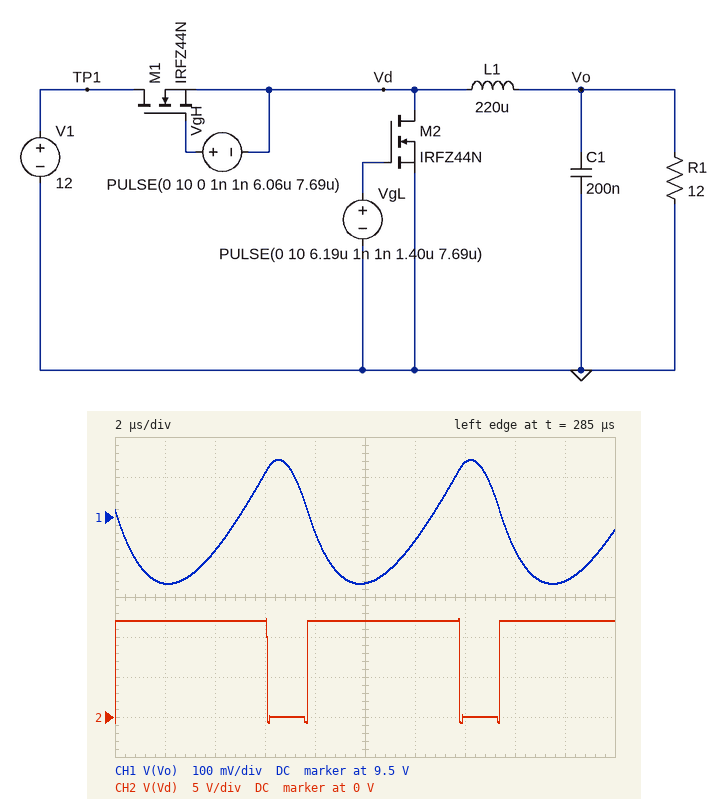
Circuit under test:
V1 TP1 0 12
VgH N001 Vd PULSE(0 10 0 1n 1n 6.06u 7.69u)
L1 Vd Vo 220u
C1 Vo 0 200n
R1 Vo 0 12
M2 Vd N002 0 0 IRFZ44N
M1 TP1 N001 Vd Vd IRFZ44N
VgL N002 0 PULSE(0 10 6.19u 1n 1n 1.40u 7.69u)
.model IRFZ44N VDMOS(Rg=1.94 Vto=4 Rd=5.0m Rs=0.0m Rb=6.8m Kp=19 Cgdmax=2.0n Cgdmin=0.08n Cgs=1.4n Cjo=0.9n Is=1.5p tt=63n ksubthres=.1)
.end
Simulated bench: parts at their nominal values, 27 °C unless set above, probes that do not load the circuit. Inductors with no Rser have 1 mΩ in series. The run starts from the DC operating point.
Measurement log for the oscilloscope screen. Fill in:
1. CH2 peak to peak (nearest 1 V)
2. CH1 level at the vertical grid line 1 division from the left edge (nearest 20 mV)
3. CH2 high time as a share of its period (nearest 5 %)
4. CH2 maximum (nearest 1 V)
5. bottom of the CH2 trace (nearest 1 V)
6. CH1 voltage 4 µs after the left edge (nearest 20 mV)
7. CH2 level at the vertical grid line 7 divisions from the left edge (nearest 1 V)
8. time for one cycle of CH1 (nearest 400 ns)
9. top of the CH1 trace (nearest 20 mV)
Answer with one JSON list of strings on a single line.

["13 V", "9.34 V", "80 %", "12 V", "-1 V", "9.42 V", "0 V", "7.6 µs", "9.64 V"]
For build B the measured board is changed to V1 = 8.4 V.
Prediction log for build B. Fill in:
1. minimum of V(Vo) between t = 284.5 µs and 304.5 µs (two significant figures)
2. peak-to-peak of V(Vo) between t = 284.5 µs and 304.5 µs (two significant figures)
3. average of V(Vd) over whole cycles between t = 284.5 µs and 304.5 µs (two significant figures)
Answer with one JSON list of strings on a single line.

["6.5 V", "220 mV", "6.6 V"]
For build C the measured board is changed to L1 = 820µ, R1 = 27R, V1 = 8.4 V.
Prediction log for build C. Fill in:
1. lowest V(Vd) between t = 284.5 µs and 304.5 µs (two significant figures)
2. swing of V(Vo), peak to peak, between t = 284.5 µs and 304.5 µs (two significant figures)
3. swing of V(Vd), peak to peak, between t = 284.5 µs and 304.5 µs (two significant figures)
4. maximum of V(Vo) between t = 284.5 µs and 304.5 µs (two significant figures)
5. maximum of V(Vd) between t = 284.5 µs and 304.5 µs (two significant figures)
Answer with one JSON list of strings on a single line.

["-670 mV", "61 mV", "9.7 V", "6.7 V", "9.0 V"]
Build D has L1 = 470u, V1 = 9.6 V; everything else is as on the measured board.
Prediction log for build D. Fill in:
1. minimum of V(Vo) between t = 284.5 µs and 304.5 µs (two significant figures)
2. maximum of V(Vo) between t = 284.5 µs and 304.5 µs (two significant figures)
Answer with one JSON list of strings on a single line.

["7.5 V", "7.6 V"]
